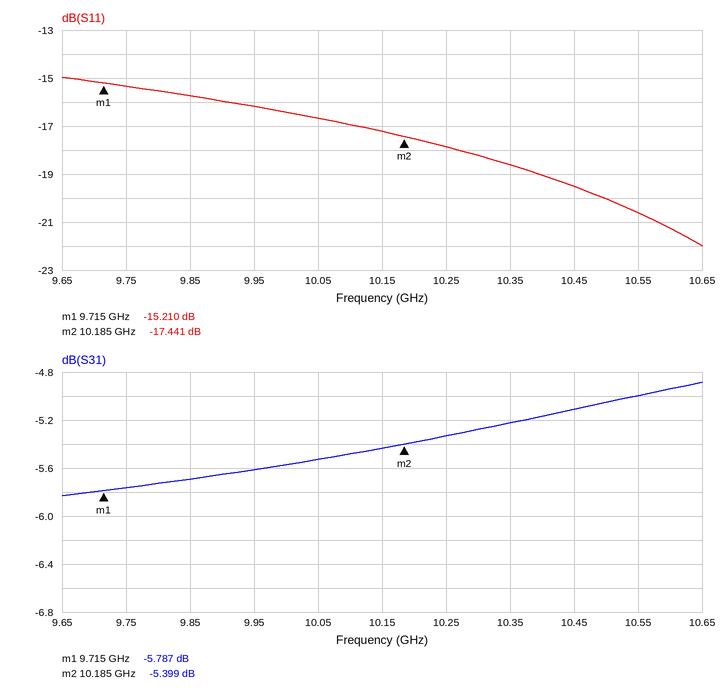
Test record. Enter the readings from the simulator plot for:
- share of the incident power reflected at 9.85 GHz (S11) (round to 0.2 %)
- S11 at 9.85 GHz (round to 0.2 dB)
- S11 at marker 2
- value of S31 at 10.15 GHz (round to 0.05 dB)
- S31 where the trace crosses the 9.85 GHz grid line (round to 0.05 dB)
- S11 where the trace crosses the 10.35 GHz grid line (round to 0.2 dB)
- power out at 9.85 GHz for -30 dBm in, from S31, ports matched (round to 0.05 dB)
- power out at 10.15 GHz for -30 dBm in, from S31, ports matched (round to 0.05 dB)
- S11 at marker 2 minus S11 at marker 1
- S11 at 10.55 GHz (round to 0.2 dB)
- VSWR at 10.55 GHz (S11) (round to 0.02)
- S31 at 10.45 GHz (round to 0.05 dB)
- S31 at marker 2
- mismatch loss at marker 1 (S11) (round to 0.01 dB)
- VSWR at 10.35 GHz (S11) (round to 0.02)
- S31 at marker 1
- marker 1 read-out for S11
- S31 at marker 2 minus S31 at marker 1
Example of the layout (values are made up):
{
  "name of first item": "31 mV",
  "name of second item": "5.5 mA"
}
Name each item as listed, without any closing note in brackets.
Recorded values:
{
  "share of the incident power reflected at 9.85 GHz (S11)": "2.6 %",
  "S11 at 9.85 GHz": "-15.8 dB",
  "S11 at marker 2": "-17.441 dB",
  "value of S31 at 10.15 GHz": "-5.45 dB",
  "S31 where the trace crosses the 9.85 GHz grid line": "-5.70 dB",
  "S11 where the trace crosses the 10.35 GHz grid line": "-18.6 dB",
  "power out at 9.85 GHz for -30 dBm in, from S31, ports matched": "-35.70 dBm",
  "power out at 10.15 GHz for -30 dBm in, from S31, ports matched": "-35.45 dBm",
  "S11 at marker 2 minus S11 at marker 1": "-2.231 dB",
  "S11 at 10.55 GHz": "-20.6 dB",
  "VSWR at 10.55 GHz (S11)": "1.20",
  "S31 at 10.45 GHz": "-5.10 dB",
  "S31 at marker 2": "-5.399 dB",
  "mismatch loss at marker 1 (S11)": "0.13 dB",
  "VSWR at 10.35 GHz (S11)": "1.26",
  "S31 at marker 1": "-5.787 dB",
  "marker 1 read-out for S11": "-15.210 dB",
  "S31 at marker 2 minus S31 at marker 1": "0.388 dB"
}
